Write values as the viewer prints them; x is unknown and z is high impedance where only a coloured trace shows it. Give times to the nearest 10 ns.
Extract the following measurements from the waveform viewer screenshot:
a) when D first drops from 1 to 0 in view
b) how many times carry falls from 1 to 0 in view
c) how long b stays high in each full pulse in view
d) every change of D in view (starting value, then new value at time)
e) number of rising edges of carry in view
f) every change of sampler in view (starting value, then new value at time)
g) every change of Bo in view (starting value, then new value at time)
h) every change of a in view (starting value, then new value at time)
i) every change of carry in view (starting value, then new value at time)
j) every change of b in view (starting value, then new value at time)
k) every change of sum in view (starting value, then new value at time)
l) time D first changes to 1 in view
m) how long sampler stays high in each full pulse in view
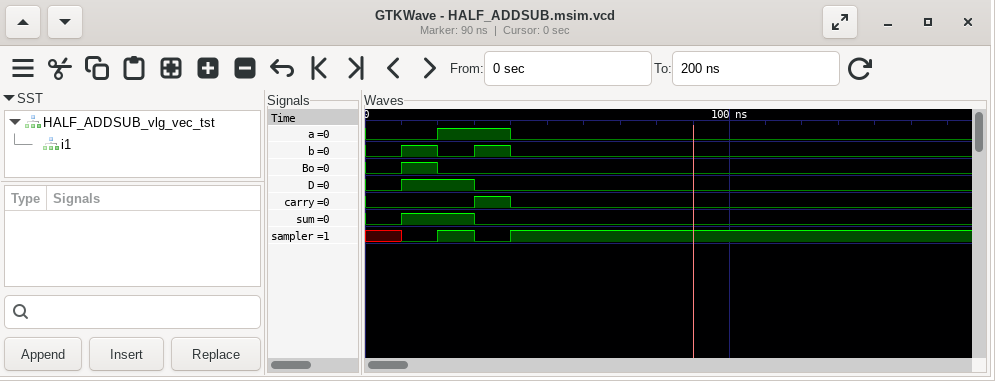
30 ns
1
10 ns, 10 ns
0, 1 at 10 ns, 0 at 30 ns
1
x, 0 at 10 ns, 1 at 20 ns, 0 at 30 ns, 1 at 40 ns
0, 1 at 10 ns, 0 at 20 ns
0, 1 at 20 ns, 0 at 40 ns
0, 1 at 30 ns, 0 at 40 ns
0, 1 at 10 ns, 0 at 20 ns, 1 at 30 ns, 0 at 40 ns
0, 1 at 10 ns, 0 at 30 ns
10 ns
10 ns
